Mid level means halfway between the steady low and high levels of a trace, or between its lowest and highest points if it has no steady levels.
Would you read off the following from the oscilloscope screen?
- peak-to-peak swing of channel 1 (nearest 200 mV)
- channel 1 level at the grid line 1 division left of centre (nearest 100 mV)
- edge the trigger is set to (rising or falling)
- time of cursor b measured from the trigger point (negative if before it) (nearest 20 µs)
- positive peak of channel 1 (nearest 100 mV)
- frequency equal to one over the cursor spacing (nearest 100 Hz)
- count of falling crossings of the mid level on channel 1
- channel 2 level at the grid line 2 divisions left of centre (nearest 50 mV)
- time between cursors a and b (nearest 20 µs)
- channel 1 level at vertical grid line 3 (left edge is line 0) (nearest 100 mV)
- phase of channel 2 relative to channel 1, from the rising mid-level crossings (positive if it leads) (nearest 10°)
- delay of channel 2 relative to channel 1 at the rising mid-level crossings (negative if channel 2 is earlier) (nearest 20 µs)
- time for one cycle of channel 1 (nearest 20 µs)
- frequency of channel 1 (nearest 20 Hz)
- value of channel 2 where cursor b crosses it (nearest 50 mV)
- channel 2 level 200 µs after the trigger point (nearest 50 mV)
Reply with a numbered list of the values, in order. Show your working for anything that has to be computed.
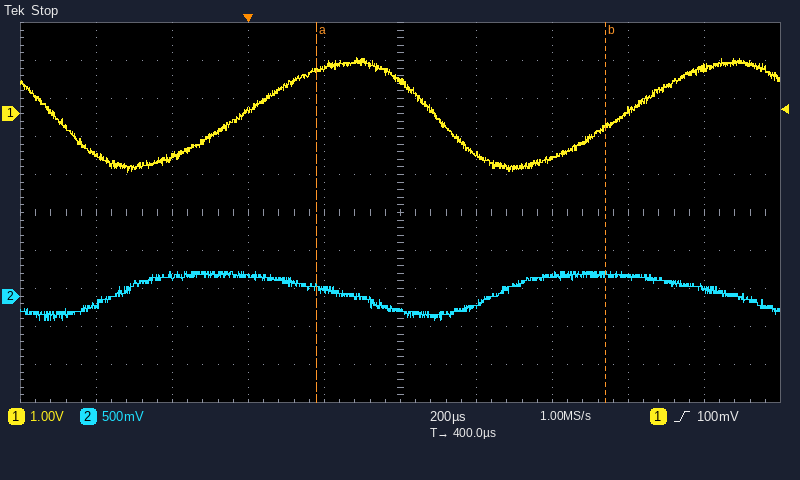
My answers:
1. 3.0 V
2. 1.2 V
3. rising
4. +940 µs
5. 1.5 V
6. 1 / 760 µs ≈ 1.3 kHz
7. 2
8. 250 mV
9. 760 µs
10. 100 mV
11. −360° × (-340 µs) / 1.00 ms ≈ +122°, so +120° to the nearest 10°
12. -340 µs
13. 1.00 ms
14. 1 / 1.00 ms ≈ 1.00 kHz
15. 300 mV
16. 100 mV
